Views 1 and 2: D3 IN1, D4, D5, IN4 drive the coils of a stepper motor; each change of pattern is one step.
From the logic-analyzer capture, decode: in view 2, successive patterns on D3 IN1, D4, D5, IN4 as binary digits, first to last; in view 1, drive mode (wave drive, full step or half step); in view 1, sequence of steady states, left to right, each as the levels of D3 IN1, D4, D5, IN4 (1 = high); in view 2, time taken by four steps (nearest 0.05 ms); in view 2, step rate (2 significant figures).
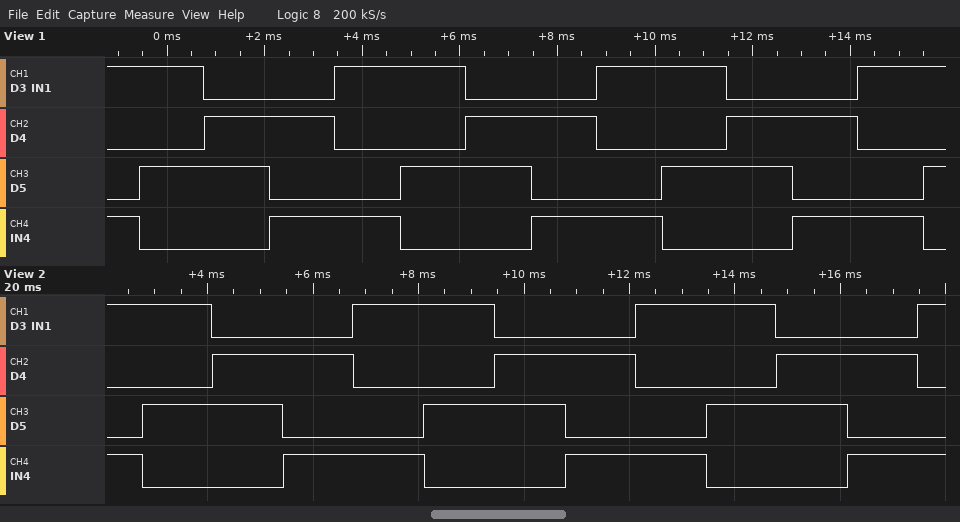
1001 1010 0110 0101 1001 1010 0110 0101 1001 1010 0110 0101 1001
full step
1001 1010 0110 0101 1001 1010 0110 0101 1001 1010 0110 0101 1001 1010
5.35 ms
750 steps/s
